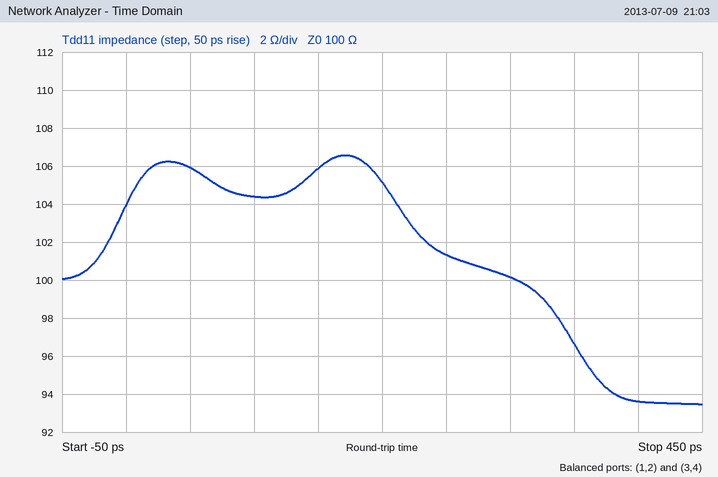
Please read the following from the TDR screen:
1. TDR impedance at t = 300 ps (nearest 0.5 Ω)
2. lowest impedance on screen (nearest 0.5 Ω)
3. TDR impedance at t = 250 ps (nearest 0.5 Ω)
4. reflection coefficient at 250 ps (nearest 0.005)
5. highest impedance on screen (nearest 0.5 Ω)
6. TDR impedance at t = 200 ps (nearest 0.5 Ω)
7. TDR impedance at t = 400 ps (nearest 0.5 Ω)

100.0 Ω
93.5 Ω
101.5 Ω
+0.005
106.5 Ω
105.0 Ω
93.5 Ω
